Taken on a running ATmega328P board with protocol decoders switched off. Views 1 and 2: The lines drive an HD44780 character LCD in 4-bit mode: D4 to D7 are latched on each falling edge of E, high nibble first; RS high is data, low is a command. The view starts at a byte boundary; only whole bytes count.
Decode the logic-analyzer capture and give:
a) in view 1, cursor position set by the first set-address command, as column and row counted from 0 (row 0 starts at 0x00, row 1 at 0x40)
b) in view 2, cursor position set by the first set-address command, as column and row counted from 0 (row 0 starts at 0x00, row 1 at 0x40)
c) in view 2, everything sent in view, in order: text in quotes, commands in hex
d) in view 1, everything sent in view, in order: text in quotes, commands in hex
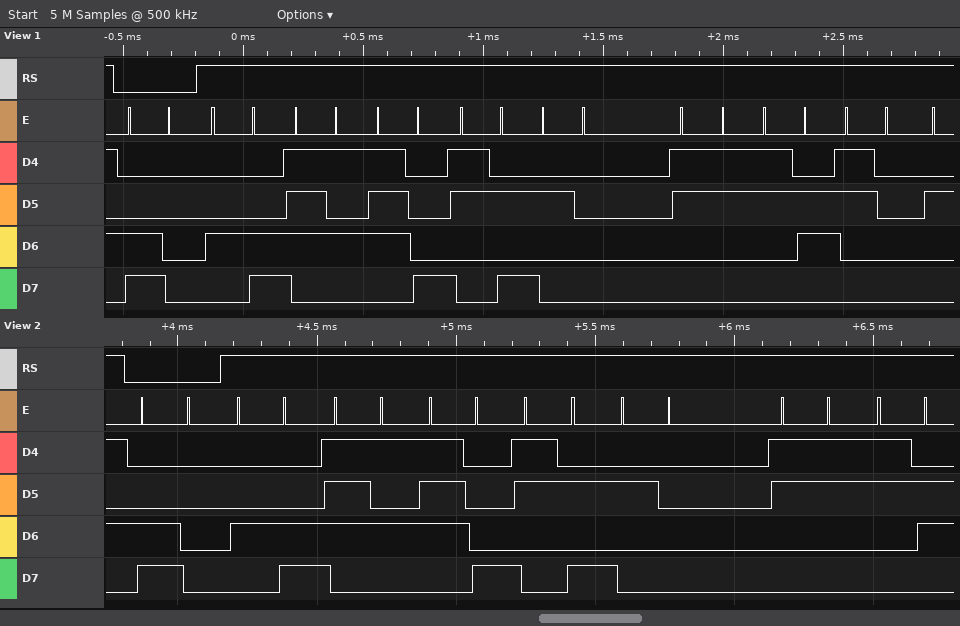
column 0, row 1
column 0, row 1
0xC0 "Lux: 36"
0xC0 "Lux: 360"
